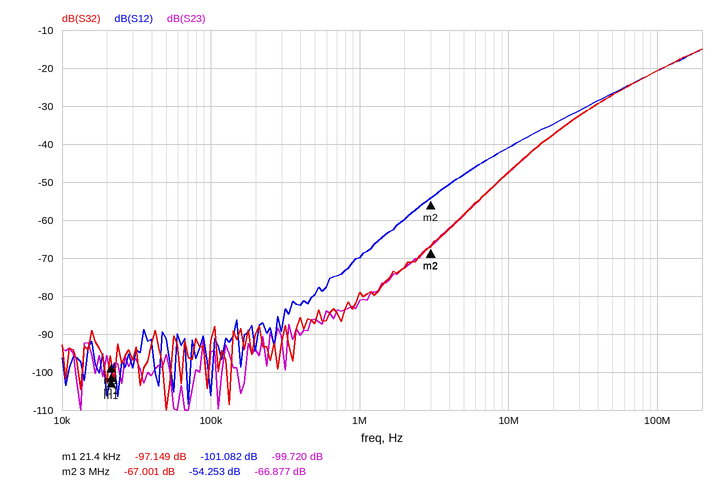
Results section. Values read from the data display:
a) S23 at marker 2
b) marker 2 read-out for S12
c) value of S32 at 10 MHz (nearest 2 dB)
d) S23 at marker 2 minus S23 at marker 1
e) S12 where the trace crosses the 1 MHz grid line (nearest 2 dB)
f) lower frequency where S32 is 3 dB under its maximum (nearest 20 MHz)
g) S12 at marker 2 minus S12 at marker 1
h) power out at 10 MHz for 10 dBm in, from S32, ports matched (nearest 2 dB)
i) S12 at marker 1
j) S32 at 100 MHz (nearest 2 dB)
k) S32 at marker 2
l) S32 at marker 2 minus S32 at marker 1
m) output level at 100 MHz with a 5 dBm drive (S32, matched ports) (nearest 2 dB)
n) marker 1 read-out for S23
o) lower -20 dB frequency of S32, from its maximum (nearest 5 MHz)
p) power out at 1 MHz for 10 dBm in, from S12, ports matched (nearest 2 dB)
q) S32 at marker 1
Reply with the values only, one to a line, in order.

-66.877 dB
-54.253 dB
-48 dB
32.843 dB
-70 dB
140 MHz
46.829 dB
-38 dBm
-101.082 dB
-20 dB
-67.001 dB
30.148 dB
-16 dBm
-99.720 dB
25 MHz
-60 dBm
-97.149 dB
